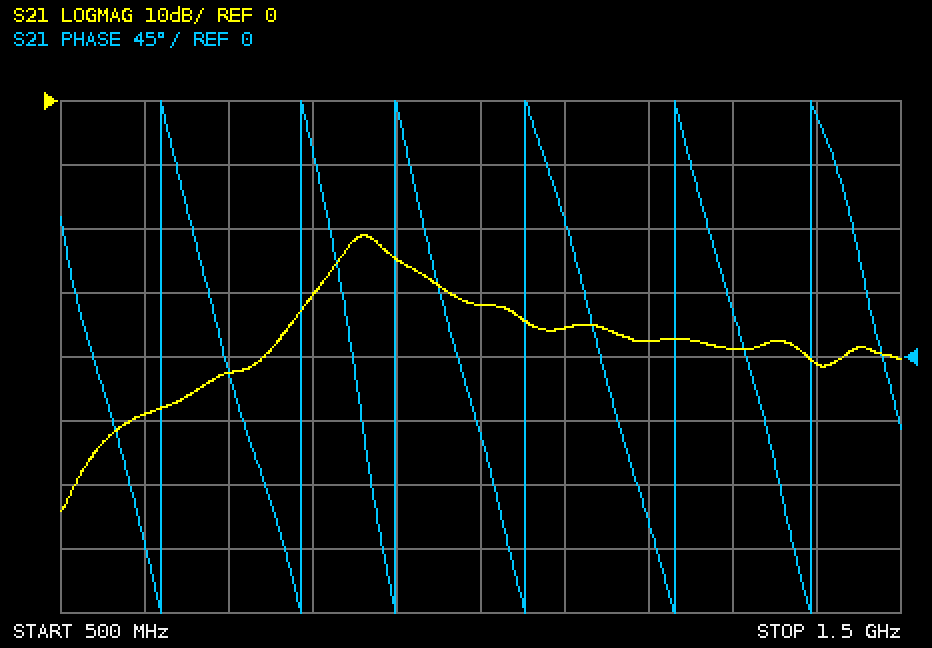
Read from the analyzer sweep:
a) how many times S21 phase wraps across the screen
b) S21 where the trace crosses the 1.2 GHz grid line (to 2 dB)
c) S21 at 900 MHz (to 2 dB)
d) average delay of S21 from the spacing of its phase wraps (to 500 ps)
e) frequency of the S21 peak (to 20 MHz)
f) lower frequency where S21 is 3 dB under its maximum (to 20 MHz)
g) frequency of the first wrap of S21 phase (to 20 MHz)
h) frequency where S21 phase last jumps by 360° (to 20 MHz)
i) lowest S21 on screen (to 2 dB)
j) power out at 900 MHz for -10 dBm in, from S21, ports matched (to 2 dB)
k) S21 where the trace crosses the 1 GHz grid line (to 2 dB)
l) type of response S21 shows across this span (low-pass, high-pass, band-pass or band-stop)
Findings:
6
-38 dB
-24 dB
6.5 ns
860 MHz
840 MHz
620 MHz
1.40 GHz
-64 dB
-34 dBm
-32 dB
band-pass
